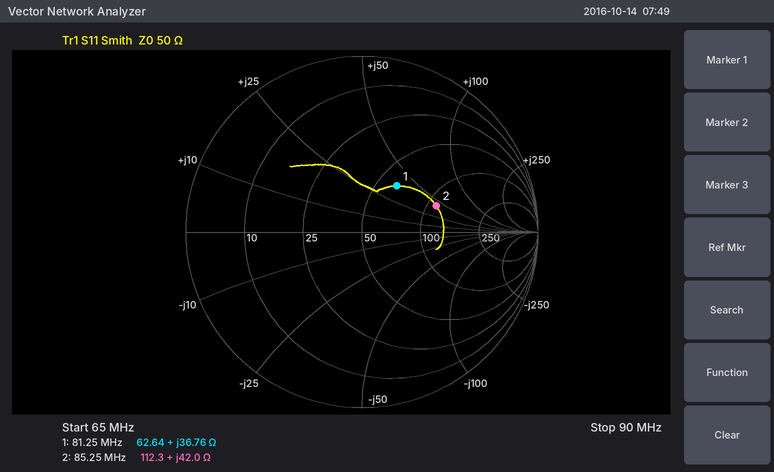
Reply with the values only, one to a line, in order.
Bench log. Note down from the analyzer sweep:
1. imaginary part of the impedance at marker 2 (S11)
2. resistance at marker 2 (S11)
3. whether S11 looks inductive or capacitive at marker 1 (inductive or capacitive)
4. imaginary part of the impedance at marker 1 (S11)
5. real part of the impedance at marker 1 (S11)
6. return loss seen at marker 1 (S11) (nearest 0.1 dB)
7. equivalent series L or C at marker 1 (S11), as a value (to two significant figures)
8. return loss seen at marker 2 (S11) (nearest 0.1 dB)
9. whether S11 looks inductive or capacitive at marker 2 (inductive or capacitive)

+42.0 Ω
112.3 Ω
inductive
+36.76 Ω
62.64 Ω
9.7 dB
72 nH
7.0 dB
inductive
